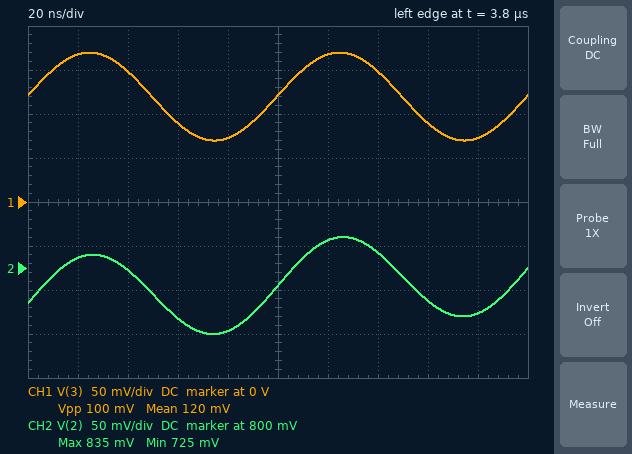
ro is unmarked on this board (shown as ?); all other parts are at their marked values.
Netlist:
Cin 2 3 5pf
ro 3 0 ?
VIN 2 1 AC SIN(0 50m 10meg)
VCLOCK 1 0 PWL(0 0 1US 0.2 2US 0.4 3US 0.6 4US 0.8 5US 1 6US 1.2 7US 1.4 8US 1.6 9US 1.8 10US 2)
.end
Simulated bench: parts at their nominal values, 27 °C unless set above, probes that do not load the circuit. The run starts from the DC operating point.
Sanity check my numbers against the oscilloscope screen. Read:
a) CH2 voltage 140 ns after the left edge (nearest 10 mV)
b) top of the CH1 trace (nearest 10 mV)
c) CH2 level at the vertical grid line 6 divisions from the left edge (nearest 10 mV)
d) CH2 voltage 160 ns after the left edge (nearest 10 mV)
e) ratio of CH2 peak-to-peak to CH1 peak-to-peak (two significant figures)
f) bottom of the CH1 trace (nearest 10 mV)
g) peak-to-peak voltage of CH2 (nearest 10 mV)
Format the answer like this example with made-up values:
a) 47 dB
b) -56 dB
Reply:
a) 820 mV
b) 170 mV
c) 830 mV
d) 760 mV
e) 1.1
f) 70 mV
g) 110 mV
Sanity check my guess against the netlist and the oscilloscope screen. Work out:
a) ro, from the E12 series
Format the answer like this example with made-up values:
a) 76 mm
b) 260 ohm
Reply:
a) 120 kΩ
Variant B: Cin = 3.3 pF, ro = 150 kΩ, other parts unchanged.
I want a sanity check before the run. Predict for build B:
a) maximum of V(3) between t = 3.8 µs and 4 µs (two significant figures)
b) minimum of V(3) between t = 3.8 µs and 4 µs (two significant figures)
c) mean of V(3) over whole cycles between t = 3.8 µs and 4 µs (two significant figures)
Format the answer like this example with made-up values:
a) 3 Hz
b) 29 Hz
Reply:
a) 150 mV
b) 49 mV
c) 99 mV
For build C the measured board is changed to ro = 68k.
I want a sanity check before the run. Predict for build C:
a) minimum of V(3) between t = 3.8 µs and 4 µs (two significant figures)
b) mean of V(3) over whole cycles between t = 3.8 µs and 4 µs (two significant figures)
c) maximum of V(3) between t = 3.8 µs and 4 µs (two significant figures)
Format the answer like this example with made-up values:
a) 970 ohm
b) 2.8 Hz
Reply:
a) 18 mV
b) 68 mV
c) 120 mV
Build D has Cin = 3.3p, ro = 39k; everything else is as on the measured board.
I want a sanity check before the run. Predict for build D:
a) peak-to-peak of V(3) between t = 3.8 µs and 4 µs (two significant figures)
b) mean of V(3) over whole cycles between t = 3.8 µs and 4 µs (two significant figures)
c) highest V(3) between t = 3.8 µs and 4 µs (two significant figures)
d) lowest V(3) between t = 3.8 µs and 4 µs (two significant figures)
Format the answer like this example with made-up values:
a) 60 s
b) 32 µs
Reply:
a) 99 mV
b) 26 mV
c) 75 mV
d) -24 mV
